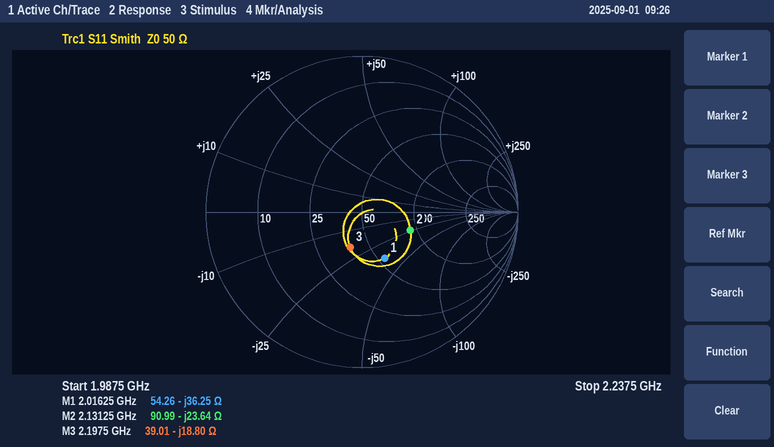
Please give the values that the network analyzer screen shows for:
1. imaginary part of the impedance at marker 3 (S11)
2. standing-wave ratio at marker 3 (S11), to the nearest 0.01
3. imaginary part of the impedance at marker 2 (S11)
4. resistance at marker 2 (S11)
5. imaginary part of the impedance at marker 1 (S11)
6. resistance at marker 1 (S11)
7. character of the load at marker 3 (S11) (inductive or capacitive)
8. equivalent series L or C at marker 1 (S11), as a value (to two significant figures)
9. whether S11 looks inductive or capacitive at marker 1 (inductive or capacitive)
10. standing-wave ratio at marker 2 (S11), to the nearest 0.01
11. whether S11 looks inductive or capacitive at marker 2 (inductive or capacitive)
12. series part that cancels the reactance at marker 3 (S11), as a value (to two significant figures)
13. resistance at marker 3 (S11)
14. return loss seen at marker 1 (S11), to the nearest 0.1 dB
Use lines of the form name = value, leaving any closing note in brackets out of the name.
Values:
imaginary part of the impedance at marker 3 = -18.80 Ω
standing-wave ratio at marker 3 (S11), to the nearest 0.01 = 1.63
imaginary part of the impedance at marker 2 = -23.64 Ω
resistance at marker 2 = 90.99 Ω
imaginary part of the impedance at marker 1 = -36.25 Ω
resistance at marker 1 = 54.26 Ω
character of the load at marker 3 (S11) = capacitive
equivalent series L or C at marker 1 (S11), as a value = 2.2 pF
whether S11 looks inductive or capacitive at marker 1 = capacitive
standing-wave ratio at marker 2 (S11), to the nearest 0.01 = 1.99
whether S11 looks inductive or capacitive at marker 2 = capacitive
series part that cancels the reactance at marker 3 (S11), as a value = 1.4 nH
resistance at marker 3 = 39.01 Ω
return loss seen at marker 1 (S11), to the nearest 0.1 dB = 9.6 dB
